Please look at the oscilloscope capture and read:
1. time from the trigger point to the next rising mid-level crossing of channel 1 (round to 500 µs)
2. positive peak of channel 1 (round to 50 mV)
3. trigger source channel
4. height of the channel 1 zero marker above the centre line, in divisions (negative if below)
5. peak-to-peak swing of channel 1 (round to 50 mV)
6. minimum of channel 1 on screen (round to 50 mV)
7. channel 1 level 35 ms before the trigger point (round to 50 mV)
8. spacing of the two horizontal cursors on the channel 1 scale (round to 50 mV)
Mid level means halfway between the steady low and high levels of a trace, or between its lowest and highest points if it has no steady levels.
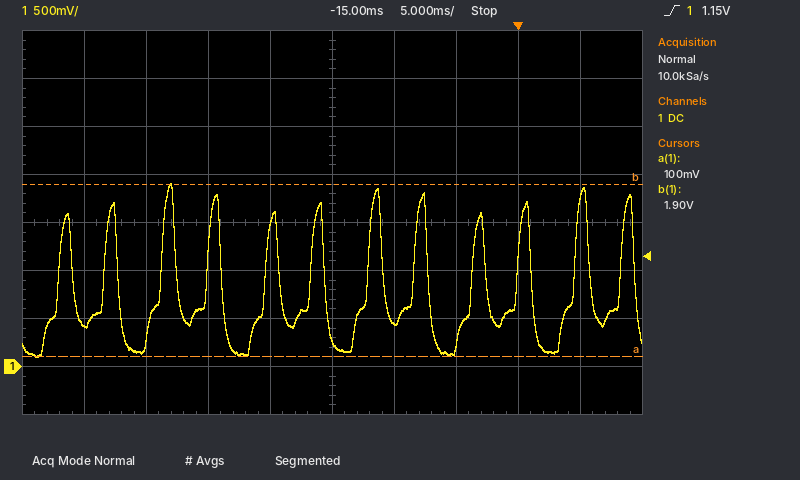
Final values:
4.5 ms
1.90 V
channel 1
-3.0 div
1.80 V
100 mV
450 mV
1.80 V
